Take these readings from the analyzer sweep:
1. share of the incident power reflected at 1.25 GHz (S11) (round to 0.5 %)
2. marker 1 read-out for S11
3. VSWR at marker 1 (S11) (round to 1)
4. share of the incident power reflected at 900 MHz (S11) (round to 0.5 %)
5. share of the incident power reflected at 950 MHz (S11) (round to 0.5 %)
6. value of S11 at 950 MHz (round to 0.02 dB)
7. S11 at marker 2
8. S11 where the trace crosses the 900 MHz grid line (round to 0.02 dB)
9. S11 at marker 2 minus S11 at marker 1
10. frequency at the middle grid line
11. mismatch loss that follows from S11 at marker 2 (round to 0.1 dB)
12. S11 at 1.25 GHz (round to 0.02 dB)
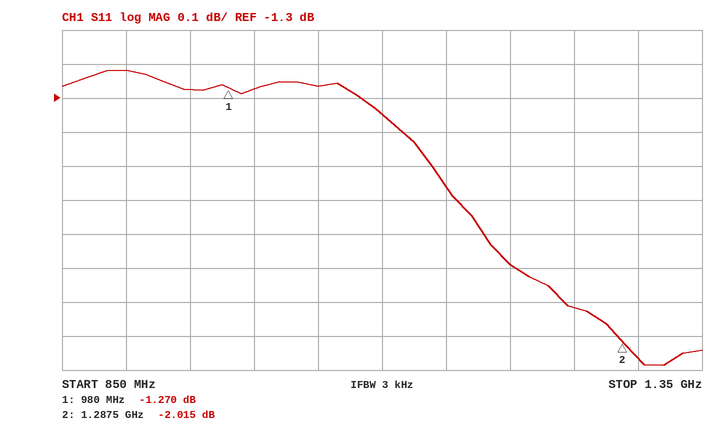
64.5 %
-1.270 dB
14
75.5 %
74.5 %
-1.28 dB
-2.015 dB
-1.22 dB
-0.745 dB
1.1 GHz
4.3 dB
-1.92 dB
